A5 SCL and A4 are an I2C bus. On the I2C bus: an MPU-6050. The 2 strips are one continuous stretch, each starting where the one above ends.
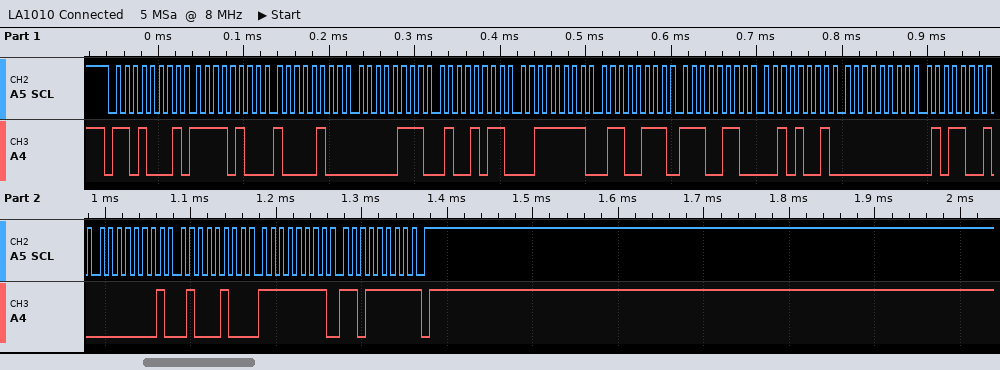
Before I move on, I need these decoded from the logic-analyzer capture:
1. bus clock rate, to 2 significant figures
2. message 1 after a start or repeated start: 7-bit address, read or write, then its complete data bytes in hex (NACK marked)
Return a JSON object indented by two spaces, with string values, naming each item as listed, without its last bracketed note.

{
  "bus clock rate, to 2 significant figures": "100 kHz",
  "message 1 after a start or repeated start: 7-bit address, read or write, then its complete data bytes in hex": "0x68 read: F4 84 07 4B 3F 67 E6 29 00 59 01 44 FF DF NACK"
}
